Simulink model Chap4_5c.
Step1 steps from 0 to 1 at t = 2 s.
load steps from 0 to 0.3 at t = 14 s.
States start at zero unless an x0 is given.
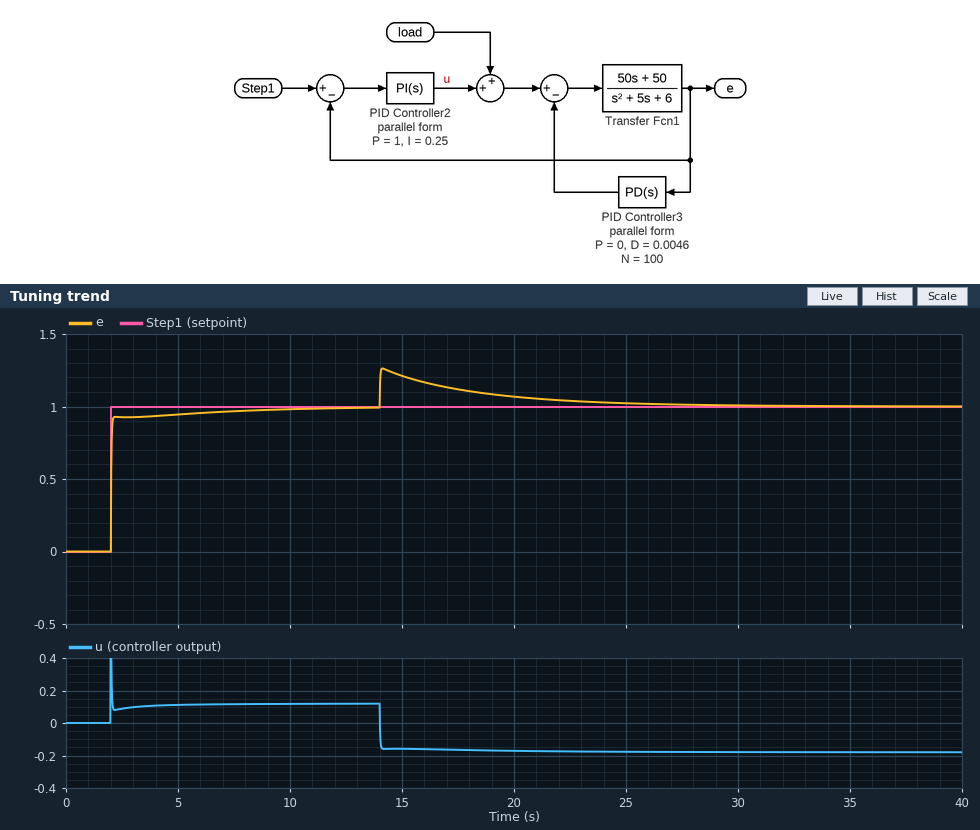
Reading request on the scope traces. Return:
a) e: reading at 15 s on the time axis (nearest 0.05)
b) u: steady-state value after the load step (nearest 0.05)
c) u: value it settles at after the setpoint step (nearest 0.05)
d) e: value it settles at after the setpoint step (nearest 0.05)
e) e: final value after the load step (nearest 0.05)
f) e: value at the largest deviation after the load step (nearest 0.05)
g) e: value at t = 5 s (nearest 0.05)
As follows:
1.20
-0.20
0.10
1.00
1.00
1.25
0.95
